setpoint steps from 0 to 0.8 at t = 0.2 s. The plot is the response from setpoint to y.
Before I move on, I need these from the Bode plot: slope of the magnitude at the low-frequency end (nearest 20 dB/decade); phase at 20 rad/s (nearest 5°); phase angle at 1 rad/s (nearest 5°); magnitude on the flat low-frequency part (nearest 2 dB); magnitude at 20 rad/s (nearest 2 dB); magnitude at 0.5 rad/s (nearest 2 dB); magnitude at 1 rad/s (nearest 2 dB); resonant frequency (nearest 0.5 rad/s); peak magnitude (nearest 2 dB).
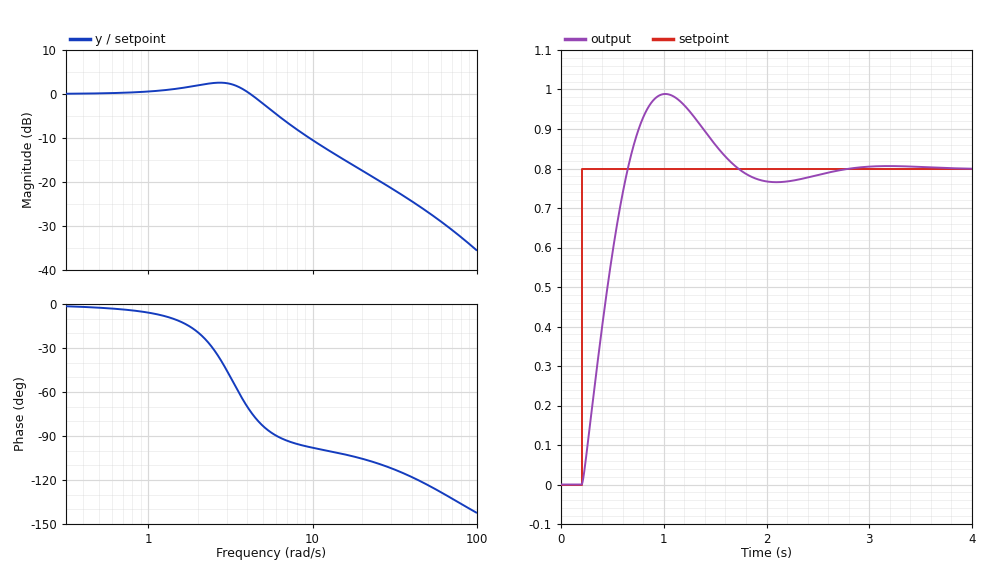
0 dB/decade
-105°
-5°
0 dB
-18 dB
0 dB
0 dB
2.5 rad/s
2 dB
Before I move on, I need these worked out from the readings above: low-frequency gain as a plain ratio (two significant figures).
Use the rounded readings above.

1.0
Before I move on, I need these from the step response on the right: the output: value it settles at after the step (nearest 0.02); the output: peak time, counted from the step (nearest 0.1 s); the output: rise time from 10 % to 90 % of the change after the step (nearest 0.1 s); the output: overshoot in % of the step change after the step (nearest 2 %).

0.80
0.8 s
0.3 s
24 %
